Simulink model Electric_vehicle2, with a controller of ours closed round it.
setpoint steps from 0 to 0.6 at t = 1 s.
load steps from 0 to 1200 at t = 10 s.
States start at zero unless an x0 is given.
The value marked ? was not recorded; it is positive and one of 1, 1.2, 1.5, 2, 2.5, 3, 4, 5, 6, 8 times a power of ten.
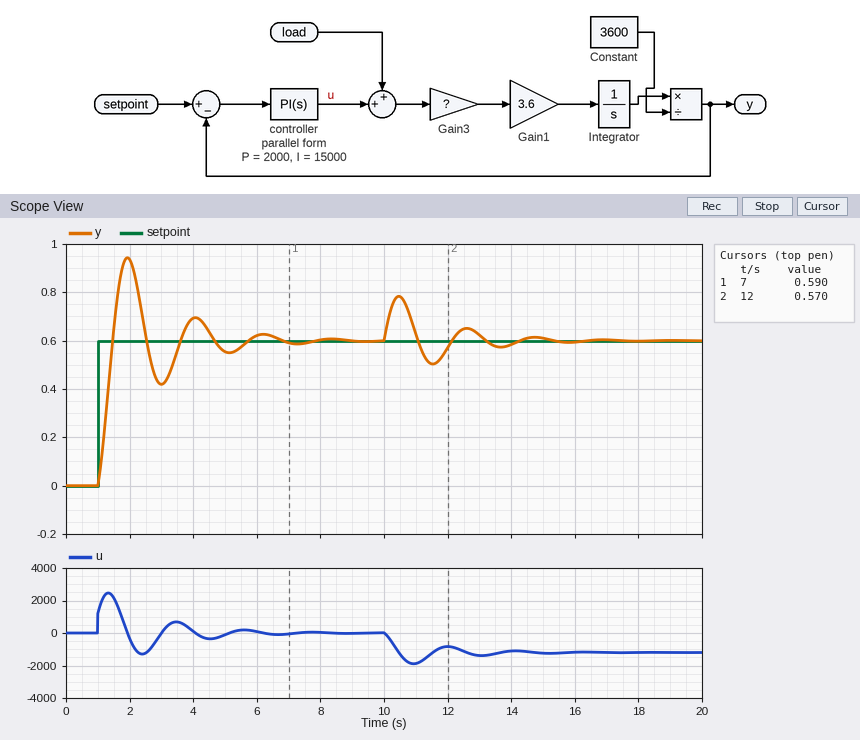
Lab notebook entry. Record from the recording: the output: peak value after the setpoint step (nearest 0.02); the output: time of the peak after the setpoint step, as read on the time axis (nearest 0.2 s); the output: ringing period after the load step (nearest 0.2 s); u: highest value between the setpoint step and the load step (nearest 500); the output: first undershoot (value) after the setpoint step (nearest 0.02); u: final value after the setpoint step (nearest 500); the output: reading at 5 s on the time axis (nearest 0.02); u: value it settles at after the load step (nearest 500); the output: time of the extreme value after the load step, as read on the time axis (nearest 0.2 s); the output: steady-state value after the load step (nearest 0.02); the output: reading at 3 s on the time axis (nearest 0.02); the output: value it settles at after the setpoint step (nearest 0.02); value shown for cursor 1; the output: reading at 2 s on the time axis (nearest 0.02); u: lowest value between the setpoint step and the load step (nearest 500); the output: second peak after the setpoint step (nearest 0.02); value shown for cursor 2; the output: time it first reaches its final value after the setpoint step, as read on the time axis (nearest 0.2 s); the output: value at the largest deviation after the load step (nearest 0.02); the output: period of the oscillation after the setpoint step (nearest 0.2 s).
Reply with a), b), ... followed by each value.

a) 0.94
b) 2.0 s
c) 2.2 s
d) 2500
e) 0.42
f) 0
g) 0.56
h) -1000
i) 10.4 s
j) 0.60
k) 0.42
l) 0.60
m) 0.590
n) 0.94
o) -1500
p) 0.70
q) 0.570
r) 1.4 s
s) 0.78
t) 2.2 s
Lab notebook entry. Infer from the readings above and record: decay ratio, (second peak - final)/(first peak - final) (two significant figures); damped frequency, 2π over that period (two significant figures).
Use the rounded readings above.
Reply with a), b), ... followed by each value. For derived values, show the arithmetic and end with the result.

a) (0.7 - 0.6) / (0.94 - 0.6) = 0.29
b) 2π / 2.2 = 2.9 rad/s
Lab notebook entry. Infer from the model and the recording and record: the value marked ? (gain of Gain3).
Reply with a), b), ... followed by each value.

a) 0.6
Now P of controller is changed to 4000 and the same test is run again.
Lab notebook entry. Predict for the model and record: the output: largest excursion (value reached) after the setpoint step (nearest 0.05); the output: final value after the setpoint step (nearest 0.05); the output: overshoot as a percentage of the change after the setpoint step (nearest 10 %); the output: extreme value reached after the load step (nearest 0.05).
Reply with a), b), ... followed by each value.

a) 0.80
b) 0.60
c) 40 %
d) 0.75
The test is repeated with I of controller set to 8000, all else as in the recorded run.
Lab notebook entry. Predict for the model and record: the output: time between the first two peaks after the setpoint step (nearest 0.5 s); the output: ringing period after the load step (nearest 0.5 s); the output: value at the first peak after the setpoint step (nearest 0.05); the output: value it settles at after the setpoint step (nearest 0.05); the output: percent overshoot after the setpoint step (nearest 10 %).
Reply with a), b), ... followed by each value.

a) 3.0 s
b) 3.0 s
c) 0.90
d) 0.60
e) 50 %
